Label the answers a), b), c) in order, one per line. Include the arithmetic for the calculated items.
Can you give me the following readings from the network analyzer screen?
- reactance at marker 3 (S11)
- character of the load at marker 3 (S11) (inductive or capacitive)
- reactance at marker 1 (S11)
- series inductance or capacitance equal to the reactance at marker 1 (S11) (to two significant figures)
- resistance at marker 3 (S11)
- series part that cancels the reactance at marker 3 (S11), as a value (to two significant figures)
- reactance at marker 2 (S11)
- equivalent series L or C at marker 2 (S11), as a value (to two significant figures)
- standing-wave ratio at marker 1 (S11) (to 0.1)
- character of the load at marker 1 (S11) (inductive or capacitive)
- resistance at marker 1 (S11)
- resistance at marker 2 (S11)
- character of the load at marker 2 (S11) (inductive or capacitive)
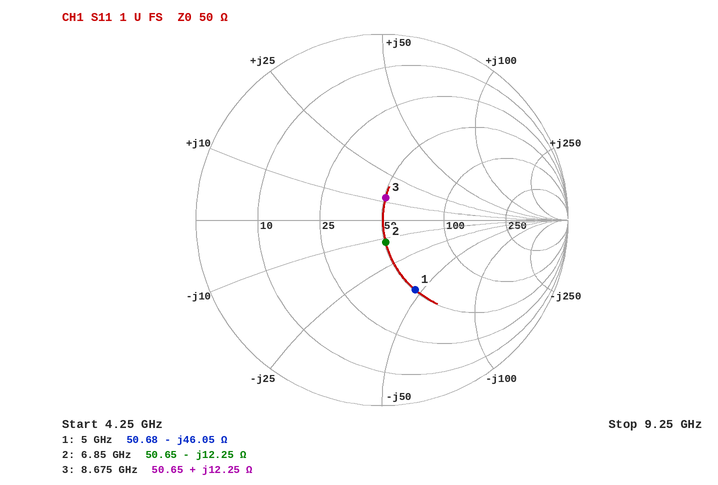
a) +12.25 Ω
b) inductive
c) -46.05 Ω
d) C = 1/(2π × 5 GHz × 46.05 Ω) ≈ 691 fF, so 690 fF to two significant figures
e) 50.65 Ω
f) C = 1/(2π × 8.675 GHz × 12.25 Ω) ≈ 1.5 pF
g) -12.25 Ω
h) C = 1/(2π × 6.85 GHz × 12.25 Ω) ≈ 1.9 pF
i) 2.4
j) capacitive
k) 50.68 Ω
l) 50.65 Ω
m) capacitive
